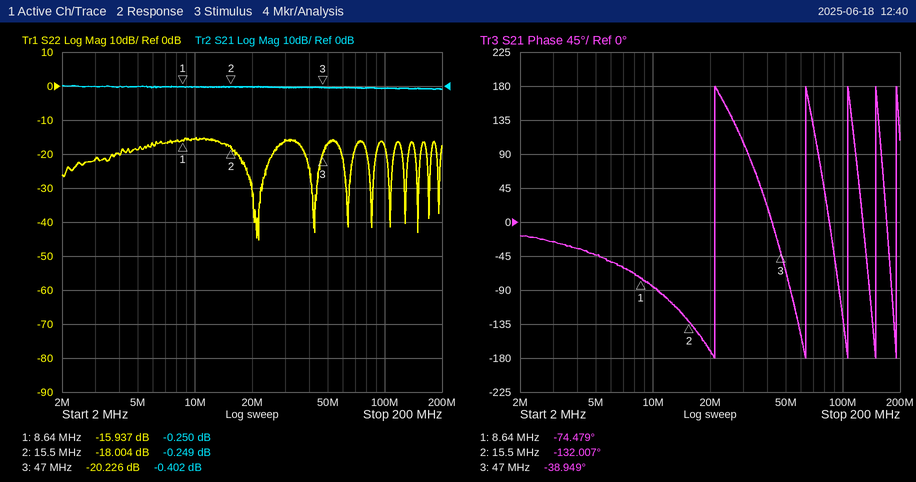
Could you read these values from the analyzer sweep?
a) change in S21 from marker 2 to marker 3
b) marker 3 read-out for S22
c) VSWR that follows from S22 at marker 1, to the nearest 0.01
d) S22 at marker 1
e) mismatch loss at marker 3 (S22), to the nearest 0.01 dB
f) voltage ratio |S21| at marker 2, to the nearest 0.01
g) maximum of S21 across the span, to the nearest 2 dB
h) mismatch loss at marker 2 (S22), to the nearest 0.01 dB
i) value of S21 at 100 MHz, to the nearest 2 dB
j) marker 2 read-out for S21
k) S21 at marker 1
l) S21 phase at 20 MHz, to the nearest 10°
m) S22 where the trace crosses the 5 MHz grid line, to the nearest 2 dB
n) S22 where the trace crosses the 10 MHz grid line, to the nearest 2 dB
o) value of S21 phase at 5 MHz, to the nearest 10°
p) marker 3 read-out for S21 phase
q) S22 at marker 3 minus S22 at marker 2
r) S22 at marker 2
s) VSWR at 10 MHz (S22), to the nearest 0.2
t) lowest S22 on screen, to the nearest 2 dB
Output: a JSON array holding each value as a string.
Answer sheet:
["-0.153 dB", "-20.226 dB", "1.38", "-15.937 dB", "0.04 dB", "0.97", "0 dB", "0.07 dB", "0 dB", "-0.249 dB", "-0.250 dB", "-170°", "-18 dB", "-16 dB", "-40°", "-38.949°", "-2.222 dB", "-18.004 dB", "1.4", "-46 dB"]
